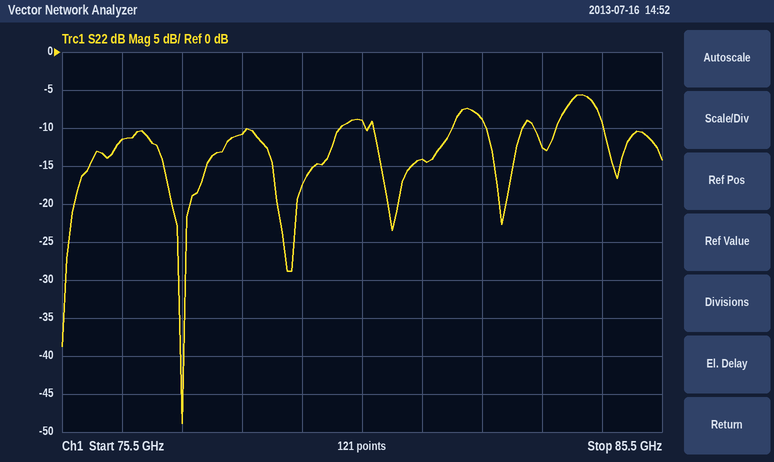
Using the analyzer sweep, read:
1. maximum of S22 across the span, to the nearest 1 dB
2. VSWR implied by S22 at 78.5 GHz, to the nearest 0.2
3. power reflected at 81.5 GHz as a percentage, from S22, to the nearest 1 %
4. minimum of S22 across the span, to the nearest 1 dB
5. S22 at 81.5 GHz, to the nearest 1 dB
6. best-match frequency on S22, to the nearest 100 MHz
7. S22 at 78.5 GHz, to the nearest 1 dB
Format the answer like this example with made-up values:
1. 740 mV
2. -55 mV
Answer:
1. -6 dB
2. 1.8
3. 4 %
4. -49 dB
5. -14 dB
6. 77.5 GHz
7. -11 dB
